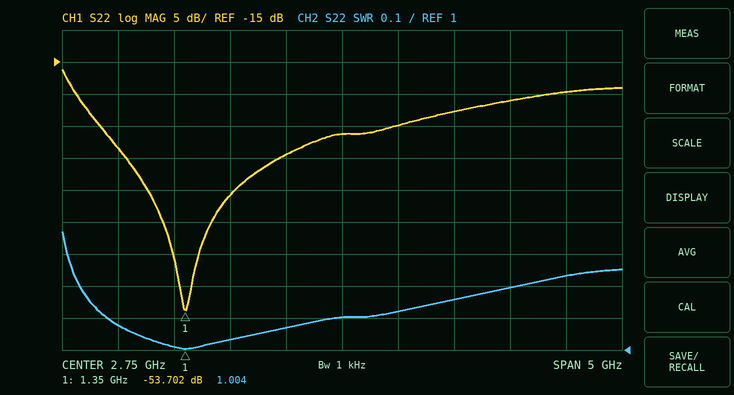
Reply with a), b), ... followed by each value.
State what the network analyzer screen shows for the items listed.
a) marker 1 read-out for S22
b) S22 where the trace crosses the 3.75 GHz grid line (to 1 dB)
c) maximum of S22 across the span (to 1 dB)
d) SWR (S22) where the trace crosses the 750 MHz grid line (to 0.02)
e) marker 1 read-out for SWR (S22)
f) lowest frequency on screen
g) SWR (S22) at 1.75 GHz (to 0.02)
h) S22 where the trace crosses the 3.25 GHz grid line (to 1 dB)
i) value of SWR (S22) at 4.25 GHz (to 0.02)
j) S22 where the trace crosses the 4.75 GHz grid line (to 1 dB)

a) -53.702 dB
b) -23 dB
c) -16 dB
d) 1.08
e) 1.004
f) 250 MHz
g) 1.04
h) -25 dB
i) 1.20
j) -20 dB
